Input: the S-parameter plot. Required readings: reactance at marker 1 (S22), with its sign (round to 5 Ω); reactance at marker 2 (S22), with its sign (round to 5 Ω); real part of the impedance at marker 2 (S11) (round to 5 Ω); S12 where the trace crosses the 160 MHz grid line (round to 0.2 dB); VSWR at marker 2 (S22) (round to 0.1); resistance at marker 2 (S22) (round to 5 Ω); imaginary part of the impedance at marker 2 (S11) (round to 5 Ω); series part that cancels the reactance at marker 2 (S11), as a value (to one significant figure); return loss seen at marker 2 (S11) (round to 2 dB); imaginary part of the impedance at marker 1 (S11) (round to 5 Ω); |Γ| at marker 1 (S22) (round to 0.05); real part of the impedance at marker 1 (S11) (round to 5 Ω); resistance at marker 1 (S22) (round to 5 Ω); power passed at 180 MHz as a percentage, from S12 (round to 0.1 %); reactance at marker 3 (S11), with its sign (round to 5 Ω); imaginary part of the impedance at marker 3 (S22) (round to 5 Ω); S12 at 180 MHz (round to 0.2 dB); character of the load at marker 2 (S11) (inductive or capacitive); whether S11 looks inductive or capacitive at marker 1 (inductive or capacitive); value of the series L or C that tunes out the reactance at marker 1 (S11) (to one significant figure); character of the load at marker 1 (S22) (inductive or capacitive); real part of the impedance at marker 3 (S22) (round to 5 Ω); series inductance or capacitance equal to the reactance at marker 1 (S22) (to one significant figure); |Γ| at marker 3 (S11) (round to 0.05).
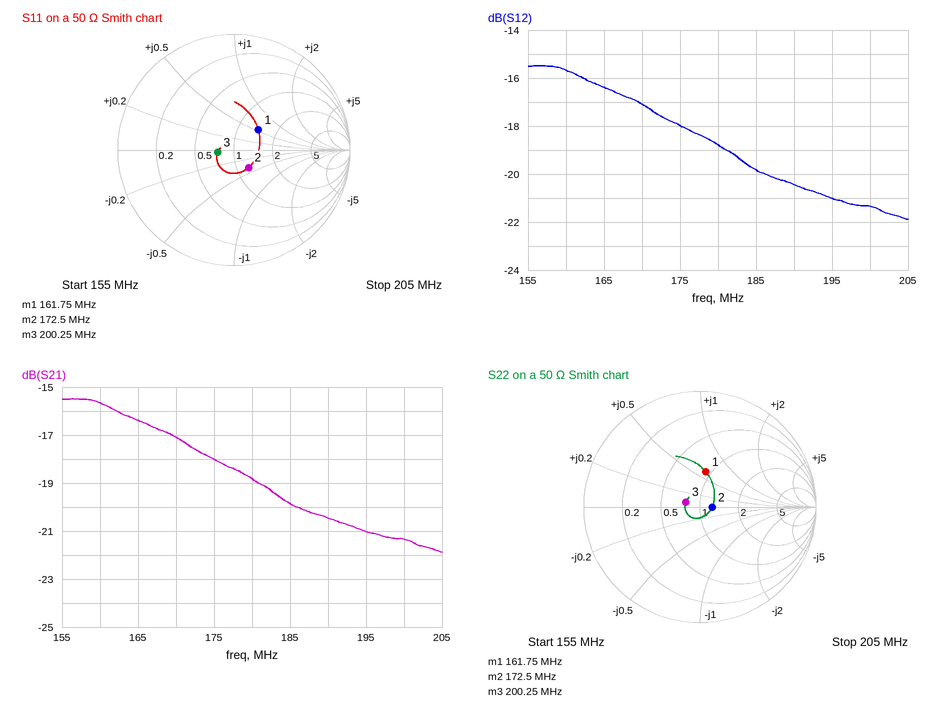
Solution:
+30 Ω
0 Ω
60 Ω
-15.6 dB
1.2
60 Ω
-20 Ω
20 nH
14 dB
+25 Ω
0.30
70 Ω
45 Ω
1.3 %
0 Ω
+5 Ω
-18.8 dB
capacitive
inductive
40 pF
inductive
40 Ω
30 nH
0.15
